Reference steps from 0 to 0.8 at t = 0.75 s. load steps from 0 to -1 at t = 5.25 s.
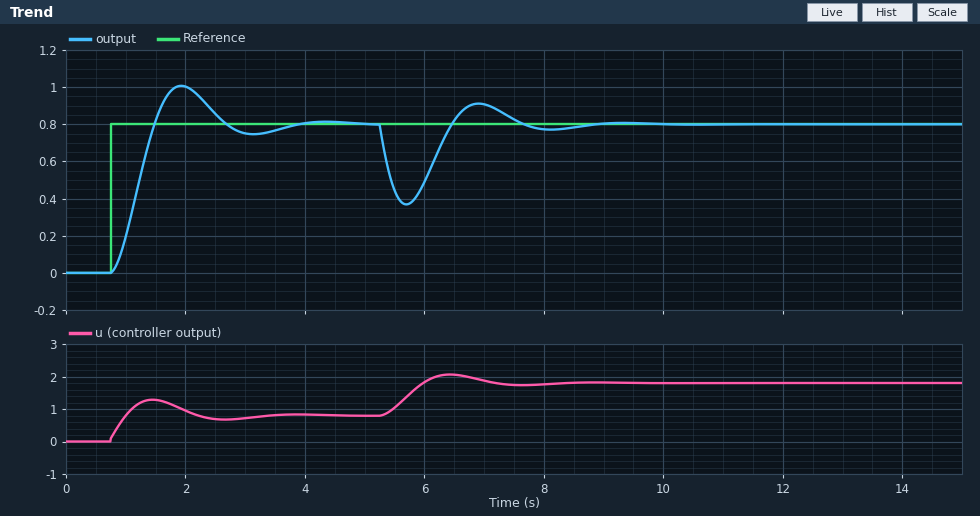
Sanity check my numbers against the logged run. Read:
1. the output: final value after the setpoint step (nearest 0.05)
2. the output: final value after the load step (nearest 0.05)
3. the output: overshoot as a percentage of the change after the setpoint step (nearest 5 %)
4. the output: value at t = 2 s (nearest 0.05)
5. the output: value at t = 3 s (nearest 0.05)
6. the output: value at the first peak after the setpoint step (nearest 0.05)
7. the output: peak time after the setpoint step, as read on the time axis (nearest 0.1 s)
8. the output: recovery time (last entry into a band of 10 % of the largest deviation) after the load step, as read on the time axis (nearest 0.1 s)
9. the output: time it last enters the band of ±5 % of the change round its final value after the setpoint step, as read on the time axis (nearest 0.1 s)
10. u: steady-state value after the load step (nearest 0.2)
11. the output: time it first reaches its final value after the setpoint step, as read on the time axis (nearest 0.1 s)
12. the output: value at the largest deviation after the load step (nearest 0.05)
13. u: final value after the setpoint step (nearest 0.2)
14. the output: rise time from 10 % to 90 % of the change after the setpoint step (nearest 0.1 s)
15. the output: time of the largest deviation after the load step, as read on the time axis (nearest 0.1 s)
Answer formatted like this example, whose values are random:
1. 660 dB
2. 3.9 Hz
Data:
1. 0.80
2. 0.80
3. 25 %
4. 1.00
5. 0.75
6. 1.00
7. 1.9 s
8. 7.4 s
9. 3.4 s
10. 1.8
11. 1.5 s
12. 0.35
13. 0.8
14. 0.5 s
15. 5.7 s
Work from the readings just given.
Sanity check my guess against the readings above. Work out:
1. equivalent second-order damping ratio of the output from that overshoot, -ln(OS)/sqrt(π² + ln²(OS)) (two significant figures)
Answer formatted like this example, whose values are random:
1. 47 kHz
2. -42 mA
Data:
1. 0.40
